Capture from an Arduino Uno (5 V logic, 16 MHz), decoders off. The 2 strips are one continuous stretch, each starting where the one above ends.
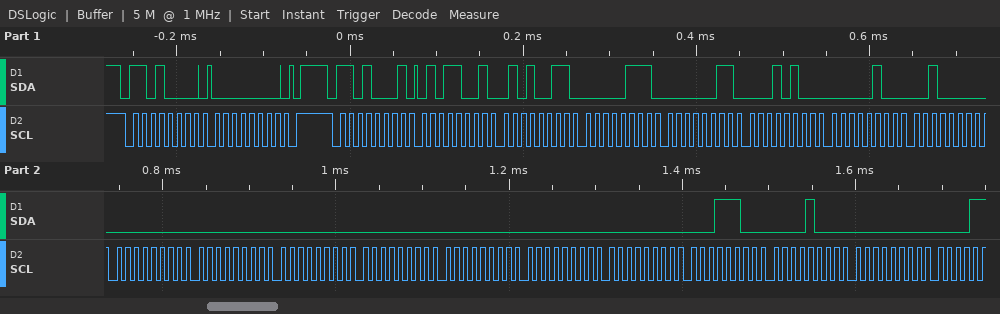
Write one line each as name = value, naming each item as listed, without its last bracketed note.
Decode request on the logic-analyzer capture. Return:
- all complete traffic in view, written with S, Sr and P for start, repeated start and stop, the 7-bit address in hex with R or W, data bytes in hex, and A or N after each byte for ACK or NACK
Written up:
all complete traffic in view, written with S, Sr and P for start, repeated start and stop, the 7-bit address in hex with R or W, data bytes in hex, and A or N after each byte for ACK or NACK = S 68W A 00 A P S 68R A 59 A 53 A 07 A 03 A 14 A 04 A 20 A 00 A 00 A 00 A 00 A 00 A 00 A 00 A 1C A 08 A 00 A
